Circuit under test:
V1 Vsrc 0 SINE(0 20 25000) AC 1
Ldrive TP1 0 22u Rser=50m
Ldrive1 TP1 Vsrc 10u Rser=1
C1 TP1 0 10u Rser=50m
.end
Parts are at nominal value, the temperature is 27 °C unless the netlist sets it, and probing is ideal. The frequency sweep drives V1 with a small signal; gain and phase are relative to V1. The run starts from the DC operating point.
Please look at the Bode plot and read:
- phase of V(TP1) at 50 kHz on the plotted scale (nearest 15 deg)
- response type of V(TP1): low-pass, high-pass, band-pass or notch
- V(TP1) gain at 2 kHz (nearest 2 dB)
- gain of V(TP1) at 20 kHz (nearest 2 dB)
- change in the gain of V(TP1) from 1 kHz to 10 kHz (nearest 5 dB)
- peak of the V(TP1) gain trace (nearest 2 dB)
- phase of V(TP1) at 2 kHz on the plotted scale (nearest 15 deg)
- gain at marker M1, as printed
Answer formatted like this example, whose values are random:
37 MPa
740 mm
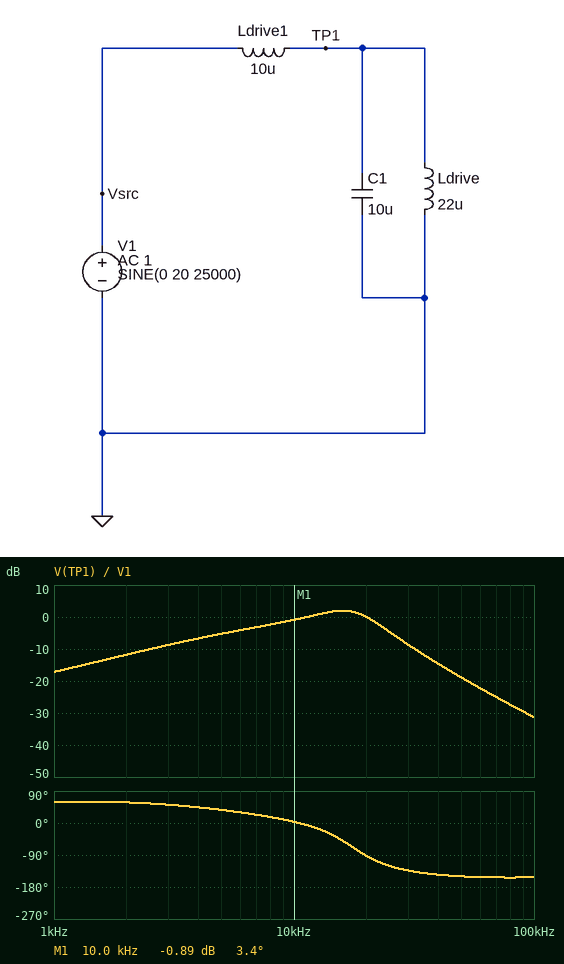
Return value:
-150 deg
band-pass
-12 dB
0 dB
15 dB
2 dB
60 deg
-0.89 dB
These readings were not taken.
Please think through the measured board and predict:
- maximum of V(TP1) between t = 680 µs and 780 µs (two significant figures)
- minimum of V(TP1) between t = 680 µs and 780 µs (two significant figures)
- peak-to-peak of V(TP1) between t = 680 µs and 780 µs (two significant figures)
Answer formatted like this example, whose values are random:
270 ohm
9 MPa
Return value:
12 V
-12 V
23 V
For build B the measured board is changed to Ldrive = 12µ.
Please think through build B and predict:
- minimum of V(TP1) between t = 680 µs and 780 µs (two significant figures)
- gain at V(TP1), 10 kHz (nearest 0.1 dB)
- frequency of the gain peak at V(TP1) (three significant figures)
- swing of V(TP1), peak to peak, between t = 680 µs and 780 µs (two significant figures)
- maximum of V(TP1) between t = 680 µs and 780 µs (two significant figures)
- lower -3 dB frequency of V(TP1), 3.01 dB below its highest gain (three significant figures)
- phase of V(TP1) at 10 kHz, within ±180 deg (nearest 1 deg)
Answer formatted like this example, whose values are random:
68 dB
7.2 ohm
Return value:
-15 V
-4.4 dB
19.2 kHz
30 V
15 V
14.2 kHz
22 deg
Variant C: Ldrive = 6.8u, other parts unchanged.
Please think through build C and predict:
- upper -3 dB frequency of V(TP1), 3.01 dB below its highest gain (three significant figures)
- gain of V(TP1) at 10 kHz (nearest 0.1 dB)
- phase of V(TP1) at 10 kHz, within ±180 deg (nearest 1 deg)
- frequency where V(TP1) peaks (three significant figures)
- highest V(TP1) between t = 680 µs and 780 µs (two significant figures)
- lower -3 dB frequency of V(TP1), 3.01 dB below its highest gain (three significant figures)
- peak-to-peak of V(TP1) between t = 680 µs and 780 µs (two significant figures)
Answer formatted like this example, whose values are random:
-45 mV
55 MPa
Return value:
27.3 kHz
-8.9 dB
33 deg
23.4 kHz
22 V
19.1 kHz
44 V
